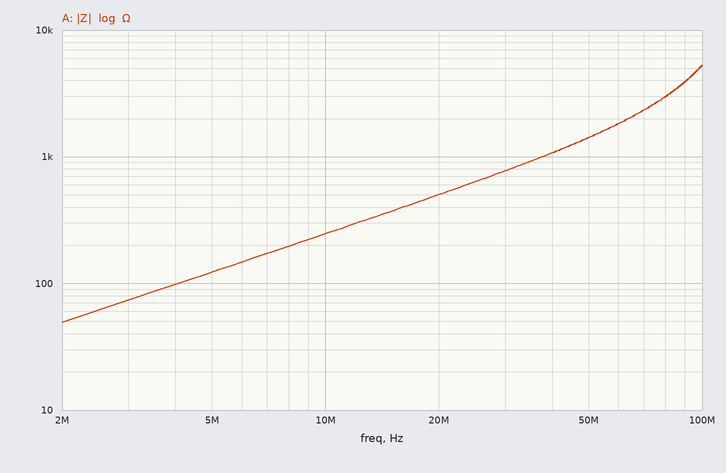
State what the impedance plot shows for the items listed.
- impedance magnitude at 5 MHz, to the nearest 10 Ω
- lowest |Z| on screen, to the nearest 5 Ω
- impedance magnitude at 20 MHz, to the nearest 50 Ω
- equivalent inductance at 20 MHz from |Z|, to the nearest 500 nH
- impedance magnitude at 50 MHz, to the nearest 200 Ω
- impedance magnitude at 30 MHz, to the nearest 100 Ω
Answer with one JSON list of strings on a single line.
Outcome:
["120 Ω", "50 Ω", "500 Ω", "4.0 µH", "1.4 kΩ", "800 Ω"]
